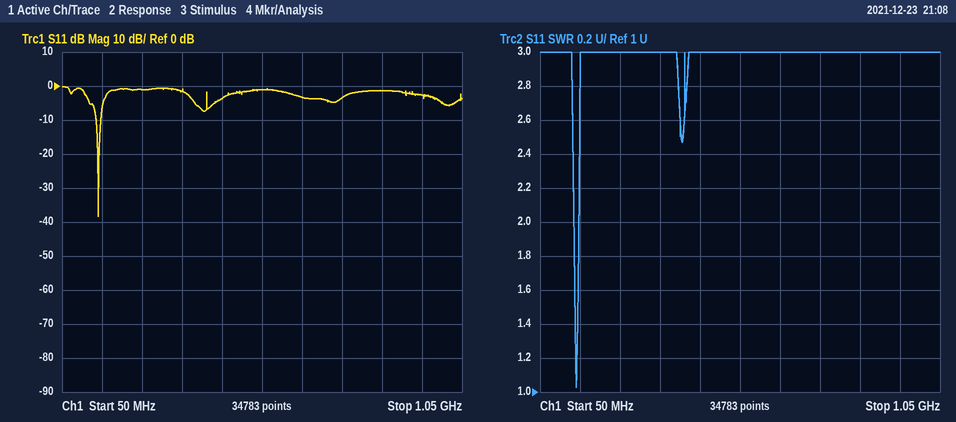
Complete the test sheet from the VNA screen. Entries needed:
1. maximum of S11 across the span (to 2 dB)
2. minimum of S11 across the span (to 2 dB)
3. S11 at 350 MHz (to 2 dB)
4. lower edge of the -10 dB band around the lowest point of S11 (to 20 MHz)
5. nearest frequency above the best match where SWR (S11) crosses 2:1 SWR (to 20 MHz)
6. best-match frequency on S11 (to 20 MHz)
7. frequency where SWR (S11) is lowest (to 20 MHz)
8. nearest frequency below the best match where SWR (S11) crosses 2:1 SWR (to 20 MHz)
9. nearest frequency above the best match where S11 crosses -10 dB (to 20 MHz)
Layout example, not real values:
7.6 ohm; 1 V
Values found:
0 dB; -38 dB; -2 dB; 140 MHz; 140 MHz; 140 MHz; 140 MHz; 140 MHz; 140 MHz
